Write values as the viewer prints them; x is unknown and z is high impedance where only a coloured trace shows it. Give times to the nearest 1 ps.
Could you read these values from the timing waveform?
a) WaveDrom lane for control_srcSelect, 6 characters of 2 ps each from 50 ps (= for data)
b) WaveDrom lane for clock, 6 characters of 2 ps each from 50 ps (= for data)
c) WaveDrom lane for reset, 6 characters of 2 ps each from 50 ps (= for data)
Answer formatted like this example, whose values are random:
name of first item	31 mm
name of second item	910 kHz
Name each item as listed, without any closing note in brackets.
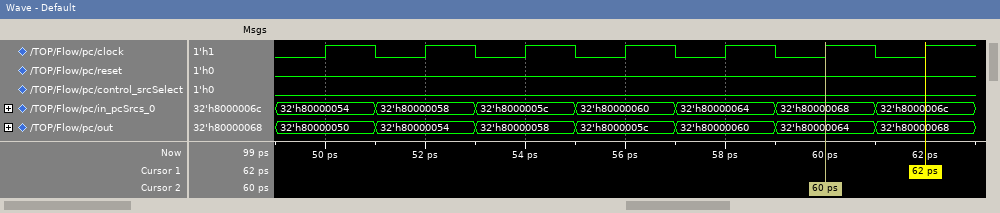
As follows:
WaveDrom lane for control_srcSelect, 6 characters of 2 ps each from 50 ps	{name: 'control_srcSelect', wave: '0.....'}
WaveDrom lane for clock, 6 characters of 2 ps each from 50 ps	{name: 'clock', wave: 'p.....'}
WaveDrom lane for reset, 6 characters of 2 ps each from 50 ps	{name: 'reset', wave: '0.....'}
